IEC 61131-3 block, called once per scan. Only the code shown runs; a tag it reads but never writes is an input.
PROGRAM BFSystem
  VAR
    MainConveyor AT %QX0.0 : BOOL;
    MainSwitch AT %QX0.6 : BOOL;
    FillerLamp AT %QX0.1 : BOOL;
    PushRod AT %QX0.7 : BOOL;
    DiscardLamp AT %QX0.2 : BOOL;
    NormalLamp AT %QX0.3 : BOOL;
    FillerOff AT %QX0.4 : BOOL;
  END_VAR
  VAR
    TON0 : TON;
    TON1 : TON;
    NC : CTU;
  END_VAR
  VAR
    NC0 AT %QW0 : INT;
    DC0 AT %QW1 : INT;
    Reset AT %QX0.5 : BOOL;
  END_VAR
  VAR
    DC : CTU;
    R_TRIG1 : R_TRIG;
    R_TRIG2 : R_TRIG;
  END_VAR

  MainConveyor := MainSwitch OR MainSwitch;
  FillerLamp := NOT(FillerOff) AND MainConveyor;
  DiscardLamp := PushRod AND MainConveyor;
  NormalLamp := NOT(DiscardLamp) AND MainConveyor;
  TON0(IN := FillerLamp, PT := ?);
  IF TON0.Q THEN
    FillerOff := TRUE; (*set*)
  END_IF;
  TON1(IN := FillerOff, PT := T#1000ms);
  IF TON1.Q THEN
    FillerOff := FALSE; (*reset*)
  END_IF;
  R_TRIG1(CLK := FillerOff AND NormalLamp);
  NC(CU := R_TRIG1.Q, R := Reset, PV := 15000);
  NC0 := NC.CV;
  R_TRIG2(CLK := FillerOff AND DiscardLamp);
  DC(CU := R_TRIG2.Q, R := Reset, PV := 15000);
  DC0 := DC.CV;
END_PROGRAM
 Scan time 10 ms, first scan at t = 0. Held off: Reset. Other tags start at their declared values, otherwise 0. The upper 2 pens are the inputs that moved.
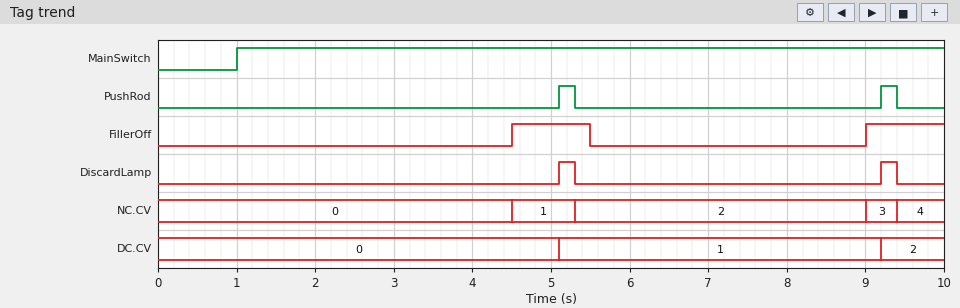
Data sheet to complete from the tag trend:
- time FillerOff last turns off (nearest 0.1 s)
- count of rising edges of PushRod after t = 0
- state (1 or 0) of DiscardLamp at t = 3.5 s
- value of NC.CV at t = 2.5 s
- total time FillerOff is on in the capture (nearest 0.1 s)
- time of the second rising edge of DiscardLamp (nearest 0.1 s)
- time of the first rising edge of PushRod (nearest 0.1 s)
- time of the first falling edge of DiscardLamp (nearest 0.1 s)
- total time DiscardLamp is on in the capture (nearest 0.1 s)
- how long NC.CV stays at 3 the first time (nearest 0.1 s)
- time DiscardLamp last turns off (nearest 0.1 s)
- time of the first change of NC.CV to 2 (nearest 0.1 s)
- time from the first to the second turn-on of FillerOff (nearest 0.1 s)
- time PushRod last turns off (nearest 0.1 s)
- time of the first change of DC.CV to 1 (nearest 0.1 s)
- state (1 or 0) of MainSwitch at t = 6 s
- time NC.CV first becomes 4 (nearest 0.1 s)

5.5 s
2
0
0
2.0 s
9.2 s
5.1 s
5.3 s
0.4 s
0.4 s
9.4 s
5.3 s
4.5 s
9.4 s
5.1 s
1
9.4 s
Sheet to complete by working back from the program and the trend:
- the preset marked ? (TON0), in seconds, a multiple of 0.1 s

3.5 s
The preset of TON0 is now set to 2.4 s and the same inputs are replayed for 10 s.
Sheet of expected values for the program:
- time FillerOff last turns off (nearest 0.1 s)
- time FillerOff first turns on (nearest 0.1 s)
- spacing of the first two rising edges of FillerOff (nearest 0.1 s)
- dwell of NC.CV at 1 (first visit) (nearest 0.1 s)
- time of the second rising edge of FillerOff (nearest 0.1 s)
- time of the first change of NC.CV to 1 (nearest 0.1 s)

7.8 s
3.4 s
3.4 s
3.4 s
6.8 s
3.4 s
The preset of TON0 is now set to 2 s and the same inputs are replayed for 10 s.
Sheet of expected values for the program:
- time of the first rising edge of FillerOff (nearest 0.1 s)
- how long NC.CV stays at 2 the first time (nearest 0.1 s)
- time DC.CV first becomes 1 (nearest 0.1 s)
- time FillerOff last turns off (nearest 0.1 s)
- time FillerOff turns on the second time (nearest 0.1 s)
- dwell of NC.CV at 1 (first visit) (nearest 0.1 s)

3.0 s
3.0 s
9.2 s
7.0 s
6.0 s
3.0 s
